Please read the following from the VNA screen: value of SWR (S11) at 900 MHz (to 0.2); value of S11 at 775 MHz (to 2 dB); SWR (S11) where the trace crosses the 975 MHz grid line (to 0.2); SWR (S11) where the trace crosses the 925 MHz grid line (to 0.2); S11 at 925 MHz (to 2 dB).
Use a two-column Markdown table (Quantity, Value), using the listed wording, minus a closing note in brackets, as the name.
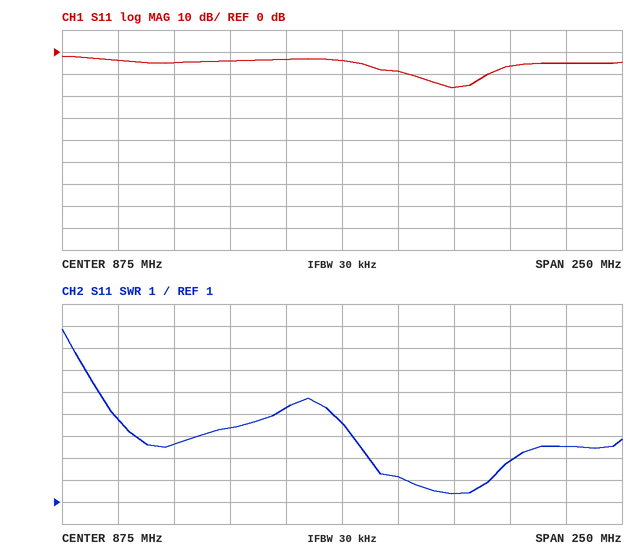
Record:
| Quantity | Value |
|---|---|
| value of SWR (S11) at 900 MHz | 2.2 |
| value of S11 at 775 MHz | -4 dB |
| SWR (S11) where the trace crosses the 975 MHz grid line | 3.6 |
| SWR (S11) where the trace crosses the 925 MHz grid line | 1.4 |
| S11 at 925 MHz | -16 dB |
